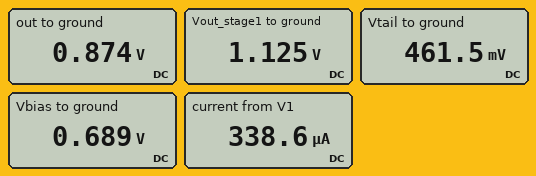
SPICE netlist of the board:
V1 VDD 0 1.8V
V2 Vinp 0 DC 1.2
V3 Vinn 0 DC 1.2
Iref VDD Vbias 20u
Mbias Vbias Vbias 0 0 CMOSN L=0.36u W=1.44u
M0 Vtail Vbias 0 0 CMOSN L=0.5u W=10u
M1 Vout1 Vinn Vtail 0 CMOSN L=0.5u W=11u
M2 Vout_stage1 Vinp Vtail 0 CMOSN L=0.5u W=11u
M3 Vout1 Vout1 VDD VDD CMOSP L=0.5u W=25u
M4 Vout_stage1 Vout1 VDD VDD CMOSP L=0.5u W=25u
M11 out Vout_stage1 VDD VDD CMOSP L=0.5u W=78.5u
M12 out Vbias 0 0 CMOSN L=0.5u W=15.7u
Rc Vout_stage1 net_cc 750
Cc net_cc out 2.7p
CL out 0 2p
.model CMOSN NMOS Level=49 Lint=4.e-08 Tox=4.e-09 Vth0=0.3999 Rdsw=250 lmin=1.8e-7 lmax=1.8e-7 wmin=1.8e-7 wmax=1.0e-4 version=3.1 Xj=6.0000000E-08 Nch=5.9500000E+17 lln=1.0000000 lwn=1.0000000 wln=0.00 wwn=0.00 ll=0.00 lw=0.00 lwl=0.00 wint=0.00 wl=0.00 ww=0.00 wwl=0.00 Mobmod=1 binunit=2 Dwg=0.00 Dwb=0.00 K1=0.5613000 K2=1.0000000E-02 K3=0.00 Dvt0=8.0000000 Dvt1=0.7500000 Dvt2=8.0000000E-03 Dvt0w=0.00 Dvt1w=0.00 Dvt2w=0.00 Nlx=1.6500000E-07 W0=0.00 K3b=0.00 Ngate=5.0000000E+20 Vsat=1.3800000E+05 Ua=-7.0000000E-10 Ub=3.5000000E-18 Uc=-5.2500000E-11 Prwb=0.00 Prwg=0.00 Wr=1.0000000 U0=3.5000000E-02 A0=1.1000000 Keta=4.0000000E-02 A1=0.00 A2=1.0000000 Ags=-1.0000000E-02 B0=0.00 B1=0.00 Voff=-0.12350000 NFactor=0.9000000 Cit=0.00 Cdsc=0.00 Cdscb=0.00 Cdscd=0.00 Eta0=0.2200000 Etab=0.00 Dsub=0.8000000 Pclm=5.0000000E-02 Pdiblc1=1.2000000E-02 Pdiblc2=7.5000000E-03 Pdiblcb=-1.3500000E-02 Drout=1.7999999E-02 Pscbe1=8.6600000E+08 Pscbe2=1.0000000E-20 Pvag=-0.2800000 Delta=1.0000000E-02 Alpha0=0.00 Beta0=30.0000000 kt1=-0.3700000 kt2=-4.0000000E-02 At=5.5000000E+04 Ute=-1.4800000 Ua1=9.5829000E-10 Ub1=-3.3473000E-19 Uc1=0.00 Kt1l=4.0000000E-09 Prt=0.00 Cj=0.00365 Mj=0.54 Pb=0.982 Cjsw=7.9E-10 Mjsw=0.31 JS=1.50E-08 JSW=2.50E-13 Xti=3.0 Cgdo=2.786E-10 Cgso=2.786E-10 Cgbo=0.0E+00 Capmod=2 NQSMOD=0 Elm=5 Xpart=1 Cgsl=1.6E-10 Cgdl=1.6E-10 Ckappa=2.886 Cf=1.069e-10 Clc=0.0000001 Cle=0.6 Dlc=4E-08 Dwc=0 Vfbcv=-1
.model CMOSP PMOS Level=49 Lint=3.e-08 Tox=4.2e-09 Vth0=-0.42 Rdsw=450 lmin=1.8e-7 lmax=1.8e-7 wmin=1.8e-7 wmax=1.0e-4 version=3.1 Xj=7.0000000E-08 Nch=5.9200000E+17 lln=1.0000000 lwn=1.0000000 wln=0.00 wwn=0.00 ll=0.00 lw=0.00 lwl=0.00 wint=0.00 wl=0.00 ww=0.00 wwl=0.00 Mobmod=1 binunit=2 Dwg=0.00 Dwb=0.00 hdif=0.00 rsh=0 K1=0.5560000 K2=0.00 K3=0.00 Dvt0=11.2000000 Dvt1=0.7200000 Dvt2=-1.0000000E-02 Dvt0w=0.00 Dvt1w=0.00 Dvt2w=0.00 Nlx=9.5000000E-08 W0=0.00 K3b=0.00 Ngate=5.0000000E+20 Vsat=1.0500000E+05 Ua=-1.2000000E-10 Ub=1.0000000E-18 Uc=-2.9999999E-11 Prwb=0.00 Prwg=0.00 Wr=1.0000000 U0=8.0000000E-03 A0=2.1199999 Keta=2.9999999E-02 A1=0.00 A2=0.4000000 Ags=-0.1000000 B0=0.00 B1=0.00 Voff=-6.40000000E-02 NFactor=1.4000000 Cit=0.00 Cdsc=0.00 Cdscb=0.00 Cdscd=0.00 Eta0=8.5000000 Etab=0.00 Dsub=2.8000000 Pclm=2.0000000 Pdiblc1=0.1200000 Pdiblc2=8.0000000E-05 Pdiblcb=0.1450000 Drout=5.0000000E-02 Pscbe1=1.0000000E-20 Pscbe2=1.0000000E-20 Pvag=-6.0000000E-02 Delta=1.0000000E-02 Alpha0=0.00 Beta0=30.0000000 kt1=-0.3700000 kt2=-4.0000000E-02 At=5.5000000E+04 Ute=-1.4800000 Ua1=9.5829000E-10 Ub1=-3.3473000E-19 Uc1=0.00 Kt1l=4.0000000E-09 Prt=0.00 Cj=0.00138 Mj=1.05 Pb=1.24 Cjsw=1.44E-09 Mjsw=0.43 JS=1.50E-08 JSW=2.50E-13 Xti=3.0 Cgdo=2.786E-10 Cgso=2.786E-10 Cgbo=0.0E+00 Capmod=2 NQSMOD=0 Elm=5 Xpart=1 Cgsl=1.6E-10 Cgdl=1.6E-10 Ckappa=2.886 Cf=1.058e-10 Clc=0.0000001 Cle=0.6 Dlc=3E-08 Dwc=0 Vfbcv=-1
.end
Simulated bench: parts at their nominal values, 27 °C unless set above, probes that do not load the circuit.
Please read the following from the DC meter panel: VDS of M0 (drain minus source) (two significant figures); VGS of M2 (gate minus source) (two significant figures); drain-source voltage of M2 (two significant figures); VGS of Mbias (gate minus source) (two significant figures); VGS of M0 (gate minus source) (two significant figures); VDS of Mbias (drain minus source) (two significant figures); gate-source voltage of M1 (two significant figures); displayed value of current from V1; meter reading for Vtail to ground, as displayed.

460 mV
740 mV
660 mV
690 mV
690 mV
690 mV
740 mV
338.6 µA
461.5 mV
